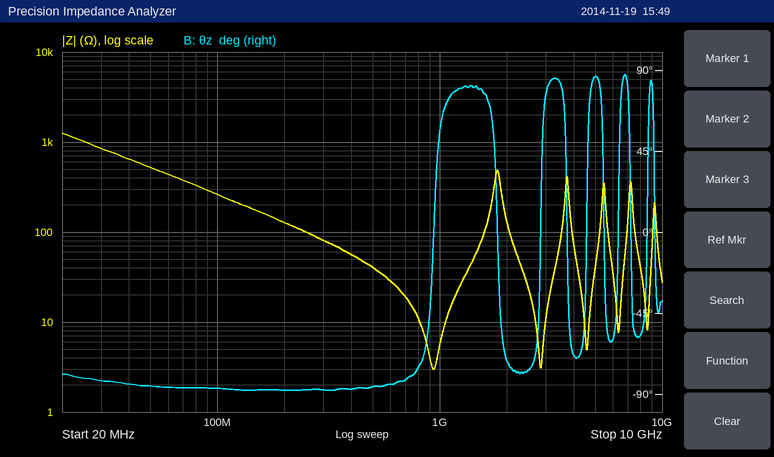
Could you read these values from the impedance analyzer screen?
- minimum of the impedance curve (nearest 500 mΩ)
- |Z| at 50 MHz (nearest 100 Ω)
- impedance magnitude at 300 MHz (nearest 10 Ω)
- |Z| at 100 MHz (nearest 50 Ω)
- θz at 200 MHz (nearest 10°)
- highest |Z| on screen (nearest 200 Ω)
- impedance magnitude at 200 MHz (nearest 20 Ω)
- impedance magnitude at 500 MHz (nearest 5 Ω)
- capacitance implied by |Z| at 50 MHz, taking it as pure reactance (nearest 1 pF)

3.0 Ω
500 Ω
80 Ω
250 Ω
-90°
1.2 kΩ
120 Ω
40 Ω
6 pF
